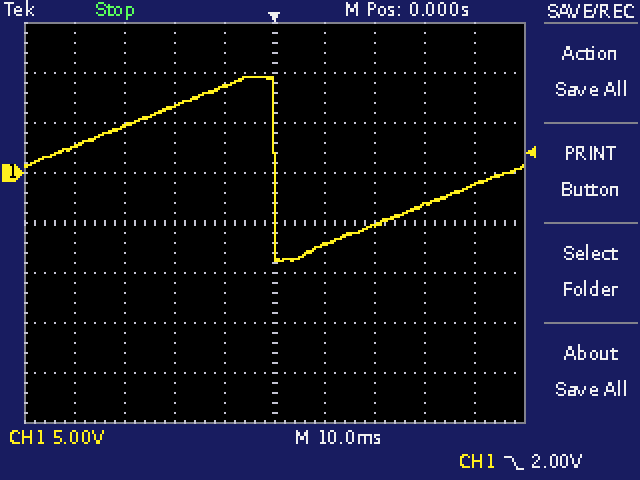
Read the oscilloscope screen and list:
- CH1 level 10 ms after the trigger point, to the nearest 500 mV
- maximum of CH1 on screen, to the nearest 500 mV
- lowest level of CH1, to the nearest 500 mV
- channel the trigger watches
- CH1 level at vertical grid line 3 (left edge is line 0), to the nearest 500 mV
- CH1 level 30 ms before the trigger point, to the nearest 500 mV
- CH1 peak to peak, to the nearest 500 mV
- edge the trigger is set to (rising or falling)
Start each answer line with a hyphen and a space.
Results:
- -7.0 V
- 9.5 V
- -9.0 V
- CH1
- 6.5 V
- 4.5 V
- 18.5 V
- falling
